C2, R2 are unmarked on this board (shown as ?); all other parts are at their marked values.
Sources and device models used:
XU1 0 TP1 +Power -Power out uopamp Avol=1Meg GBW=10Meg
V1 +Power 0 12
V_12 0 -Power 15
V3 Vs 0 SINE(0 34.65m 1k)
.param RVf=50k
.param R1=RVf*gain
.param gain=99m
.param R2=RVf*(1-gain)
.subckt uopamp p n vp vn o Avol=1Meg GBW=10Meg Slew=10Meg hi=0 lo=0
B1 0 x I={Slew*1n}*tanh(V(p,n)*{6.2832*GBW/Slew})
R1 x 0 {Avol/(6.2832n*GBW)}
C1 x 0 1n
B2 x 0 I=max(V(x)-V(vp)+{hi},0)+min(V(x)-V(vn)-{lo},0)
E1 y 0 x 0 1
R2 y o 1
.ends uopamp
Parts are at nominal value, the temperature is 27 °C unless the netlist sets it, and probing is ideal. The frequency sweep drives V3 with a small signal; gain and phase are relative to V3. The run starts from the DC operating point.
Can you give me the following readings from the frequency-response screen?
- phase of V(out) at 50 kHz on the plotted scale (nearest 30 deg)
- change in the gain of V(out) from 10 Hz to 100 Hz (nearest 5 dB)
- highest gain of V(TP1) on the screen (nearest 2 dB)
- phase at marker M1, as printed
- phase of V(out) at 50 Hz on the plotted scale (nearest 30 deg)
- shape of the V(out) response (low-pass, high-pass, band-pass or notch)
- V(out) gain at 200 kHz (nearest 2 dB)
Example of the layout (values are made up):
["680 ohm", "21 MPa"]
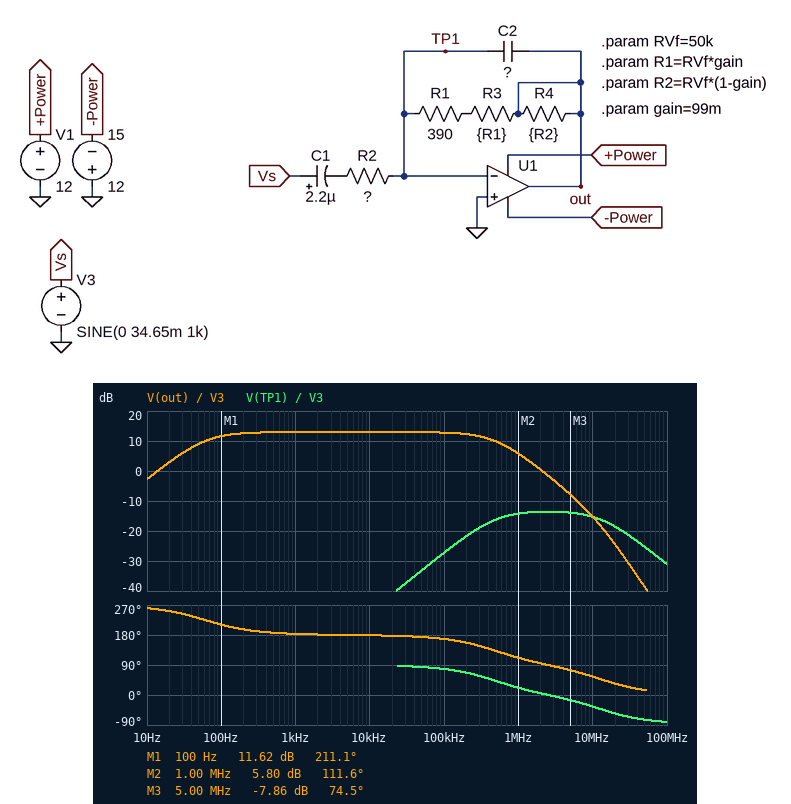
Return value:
["180 deg", "15 dB", "-14 dB", "211.1 deg", "240 deg", "band-pass", "12 dB"]
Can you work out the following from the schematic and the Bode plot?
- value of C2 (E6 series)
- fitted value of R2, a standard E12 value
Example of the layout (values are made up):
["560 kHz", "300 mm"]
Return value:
["47 pF", "1.2 kΩ"]
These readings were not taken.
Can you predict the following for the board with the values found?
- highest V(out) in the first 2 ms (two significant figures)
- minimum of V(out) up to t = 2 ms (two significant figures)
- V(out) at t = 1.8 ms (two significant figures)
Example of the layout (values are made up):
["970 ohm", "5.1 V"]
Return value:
["160 mV", "-150 mV", "150 mV"]
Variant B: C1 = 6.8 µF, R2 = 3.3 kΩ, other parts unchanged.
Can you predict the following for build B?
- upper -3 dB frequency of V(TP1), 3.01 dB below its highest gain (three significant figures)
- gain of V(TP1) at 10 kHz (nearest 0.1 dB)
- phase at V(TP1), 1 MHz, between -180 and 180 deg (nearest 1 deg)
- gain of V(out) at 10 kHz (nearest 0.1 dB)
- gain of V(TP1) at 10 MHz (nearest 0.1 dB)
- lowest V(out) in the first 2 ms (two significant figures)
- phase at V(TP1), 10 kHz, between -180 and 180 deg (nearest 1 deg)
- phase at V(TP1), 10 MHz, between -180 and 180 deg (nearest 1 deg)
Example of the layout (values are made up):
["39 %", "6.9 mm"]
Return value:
["12.2 MHz", "-55.8 dB", "25 deg", "4.2 dB", "-23.3 dB", "-56 mV", "89 deg", "-39 deg"]
